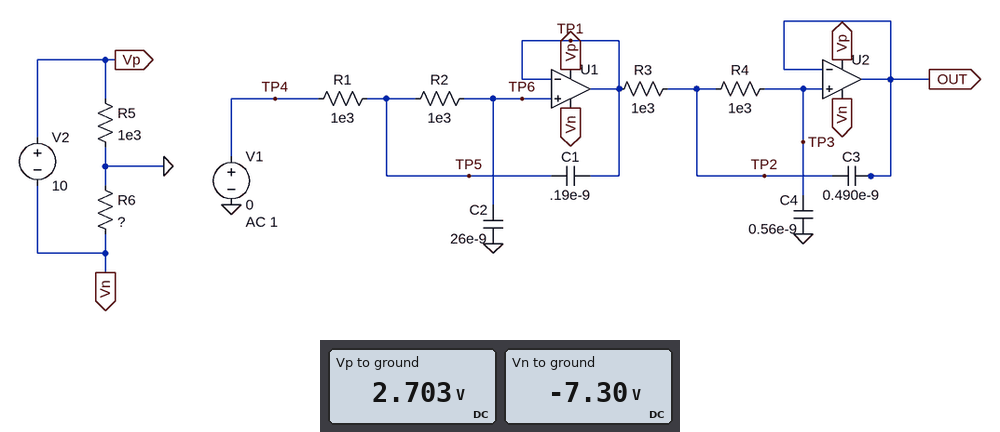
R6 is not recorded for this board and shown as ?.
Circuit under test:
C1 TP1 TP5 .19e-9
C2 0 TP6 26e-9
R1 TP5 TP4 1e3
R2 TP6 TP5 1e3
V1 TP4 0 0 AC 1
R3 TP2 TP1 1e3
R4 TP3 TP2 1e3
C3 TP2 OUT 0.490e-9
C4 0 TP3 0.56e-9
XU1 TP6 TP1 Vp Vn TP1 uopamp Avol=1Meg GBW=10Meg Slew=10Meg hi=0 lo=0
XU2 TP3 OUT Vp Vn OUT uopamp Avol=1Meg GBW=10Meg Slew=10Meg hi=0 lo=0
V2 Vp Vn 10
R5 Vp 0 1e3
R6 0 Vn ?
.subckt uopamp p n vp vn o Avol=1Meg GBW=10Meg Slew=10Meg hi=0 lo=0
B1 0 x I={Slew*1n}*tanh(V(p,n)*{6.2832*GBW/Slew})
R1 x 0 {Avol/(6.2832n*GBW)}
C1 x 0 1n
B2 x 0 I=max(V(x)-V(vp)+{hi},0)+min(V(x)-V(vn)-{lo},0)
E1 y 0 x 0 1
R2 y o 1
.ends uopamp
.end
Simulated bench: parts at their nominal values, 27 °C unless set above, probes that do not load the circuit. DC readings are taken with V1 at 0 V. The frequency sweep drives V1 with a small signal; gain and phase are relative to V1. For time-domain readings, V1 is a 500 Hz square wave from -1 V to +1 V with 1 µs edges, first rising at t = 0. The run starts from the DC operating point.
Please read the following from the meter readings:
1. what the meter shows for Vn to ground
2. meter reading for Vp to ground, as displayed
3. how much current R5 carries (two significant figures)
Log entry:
-7.30 V
2.703 V
2.7 mA
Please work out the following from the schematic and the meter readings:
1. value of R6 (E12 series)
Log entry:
2.7 kΩ
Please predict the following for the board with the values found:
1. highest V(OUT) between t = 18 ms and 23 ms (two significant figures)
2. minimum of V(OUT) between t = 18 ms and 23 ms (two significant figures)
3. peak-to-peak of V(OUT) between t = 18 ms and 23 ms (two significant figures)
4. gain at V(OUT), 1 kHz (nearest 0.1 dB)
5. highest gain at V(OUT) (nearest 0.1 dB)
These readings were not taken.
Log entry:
1.0 V
-1.0 V
2.0 V
-0.4 dB
0 dB
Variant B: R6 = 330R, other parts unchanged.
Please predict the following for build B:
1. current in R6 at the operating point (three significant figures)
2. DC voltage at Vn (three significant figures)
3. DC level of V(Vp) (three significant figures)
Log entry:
7.52 mA
-2.48 V
7.52 V
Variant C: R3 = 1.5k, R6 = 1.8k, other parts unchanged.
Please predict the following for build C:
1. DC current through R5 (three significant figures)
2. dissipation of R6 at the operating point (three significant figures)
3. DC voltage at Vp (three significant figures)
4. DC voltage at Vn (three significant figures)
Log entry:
3.57 mA
23.0 mW
3.57 V
-6.43 V
